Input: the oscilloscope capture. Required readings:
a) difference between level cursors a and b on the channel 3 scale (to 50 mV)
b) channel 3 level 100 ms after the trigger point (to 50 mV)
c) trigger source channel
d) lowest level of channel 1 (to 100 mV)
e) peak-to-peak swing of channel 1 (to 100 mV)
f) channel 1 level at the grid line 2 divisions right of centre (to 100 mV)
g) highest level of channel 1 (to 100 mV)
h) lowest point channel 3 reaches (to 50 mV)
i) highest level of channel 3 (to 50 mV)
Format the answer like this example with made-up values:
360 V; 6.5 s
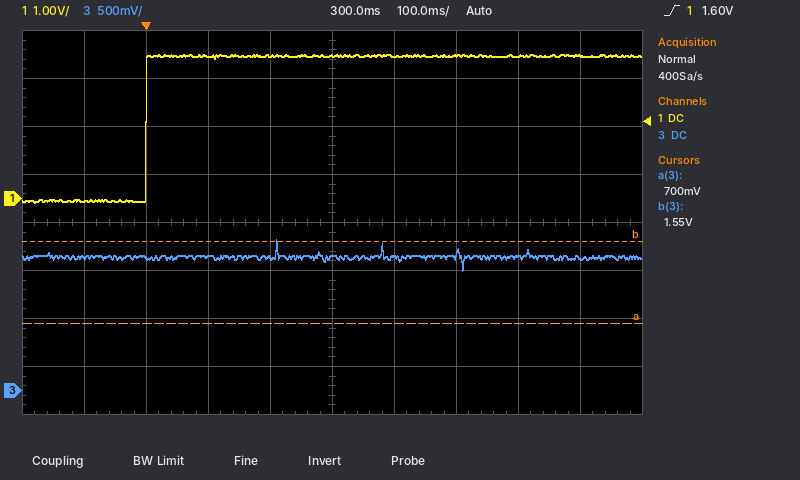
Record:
850 mV; 1.40 V; channel 1; -100 mV; 3.1 V; 3.0 V; 3.0 V; 1.25 V; 1.55 V
